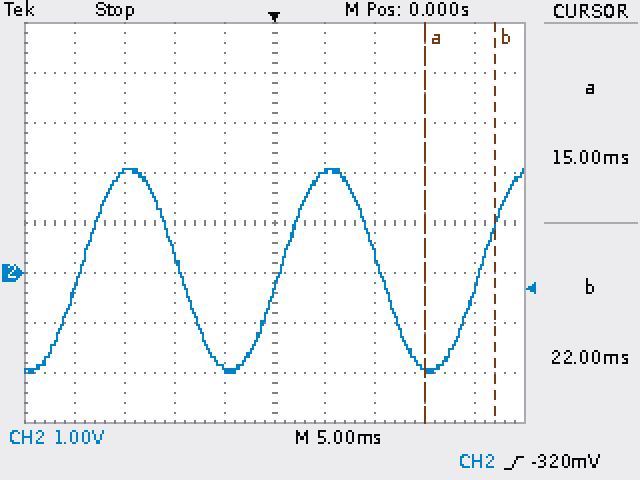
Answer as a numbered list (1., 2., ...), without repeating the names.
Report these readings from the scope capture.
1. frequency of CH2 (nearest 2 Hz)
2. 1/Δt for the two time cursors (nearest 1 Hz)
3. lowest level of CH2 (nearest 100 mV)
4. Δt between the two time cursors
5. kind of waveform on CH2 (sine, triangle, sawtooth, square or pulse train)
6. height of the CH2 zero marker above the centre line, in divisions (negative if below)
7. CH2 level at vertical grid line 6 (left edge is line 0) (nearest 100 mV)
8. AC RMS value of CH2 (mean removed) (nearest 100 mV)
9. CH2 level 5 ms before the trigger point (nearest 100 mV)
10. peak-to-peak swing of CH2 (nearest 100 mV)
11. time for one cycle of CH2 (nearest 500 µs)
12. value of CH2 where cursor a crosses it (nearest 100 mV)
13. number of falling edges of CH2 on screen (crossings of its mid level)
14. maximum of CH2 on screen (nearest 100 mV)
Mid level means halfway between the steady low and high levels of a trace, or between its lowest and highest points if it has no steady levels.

1. 50 Hz
2. 143 Hz
3. -2.0 V
4. 7.0 ms
5. sine
6. -1.0 div
7. 2.0 V
8. 1.4 V
9. -1.9 V
10. 4.1 V
11. 20.0 ms
12. -1.9 V
13. 2
14. 2.1 V
